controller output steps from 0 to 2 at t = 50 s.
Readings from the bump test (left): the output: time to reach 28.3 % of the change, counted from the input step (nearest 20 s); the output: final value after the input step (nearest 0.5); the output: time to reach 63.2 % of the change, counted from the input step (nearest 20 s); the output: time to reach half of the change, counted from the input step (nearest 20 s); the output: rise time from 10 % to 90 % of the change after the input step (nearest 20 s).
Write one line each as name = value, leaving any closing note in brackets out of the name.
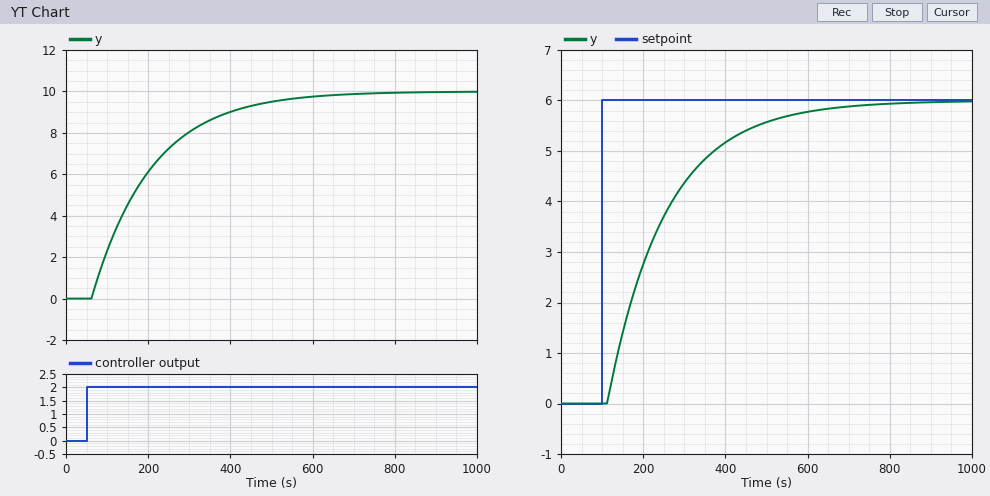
the output: time to reach 28.3 % of the change, counted from the input step = 60 s
the output: final value after the input step = 10.0
the output: time to reach 63.2 % of the change, counted from the input step = 160 s
the output: time to reach half of the change, counted from the input step = 120 s
the output: rise time from 10 % to 90 % of the change after the input step = 320 s
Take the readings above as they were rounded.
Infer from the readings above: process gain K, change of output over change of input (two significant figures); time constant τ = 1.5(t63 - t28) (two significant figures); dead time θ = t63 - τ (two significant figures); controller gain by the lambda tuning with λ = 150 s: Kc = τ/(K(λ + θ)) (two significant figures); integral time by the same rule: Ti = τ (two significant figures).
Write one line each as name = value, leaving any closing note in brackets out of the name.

process gain K, change of output over change of input = 5.0
time constant τ = 1.5(t63 - t28) = 150 s
dead time θ = t63 - τ = 10 s
controller gain by the lambda tuning with λ = 150 s: Kc = τ/(K(λ + θ)) = 0.19
integral time by the same rule: Ti = τ = 150 s
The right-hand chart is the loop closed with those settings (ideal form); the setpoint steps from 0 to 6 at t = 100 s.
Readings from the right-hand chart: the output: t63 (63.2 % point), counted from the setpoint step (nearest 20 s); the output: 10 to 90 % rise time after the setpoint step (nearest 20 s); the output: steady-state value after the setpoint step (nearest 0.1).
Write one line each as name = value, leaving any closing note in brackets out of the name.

the output: t63 (63.2 % point), counted from the setpoint step = 160 s
the output: 10 to 90 % rise time after the setpoint step = 320 s
the output: steady-state value after the setpoint step = 6.0
